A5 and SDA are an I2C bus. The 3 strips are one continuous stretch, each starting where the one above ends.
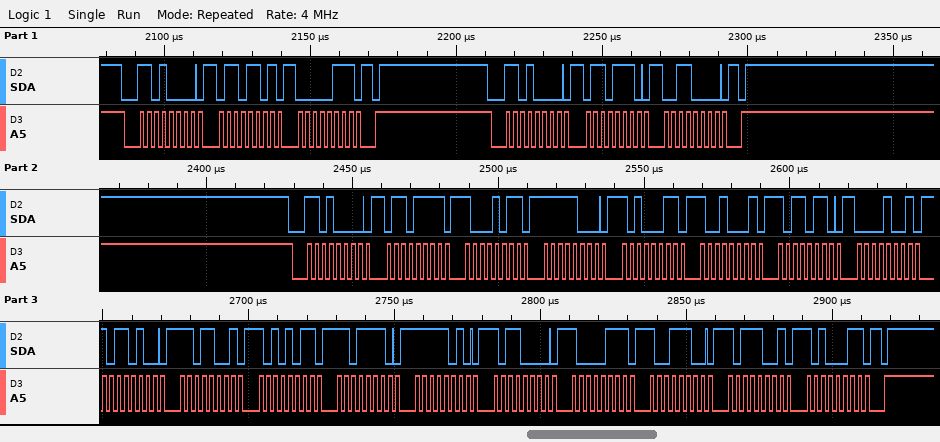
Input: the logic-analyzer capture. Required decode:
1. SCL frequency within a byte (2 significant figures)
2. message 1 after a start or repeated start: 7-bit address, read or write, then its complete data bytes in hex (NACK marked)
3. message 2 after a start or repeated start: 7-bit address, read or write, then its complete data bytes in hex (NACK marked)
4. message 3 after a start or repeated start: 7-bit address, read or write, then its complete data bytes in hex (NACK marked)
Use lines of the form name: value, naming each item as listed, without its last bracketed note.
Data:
SCL frequency within a byte: 400 kHz
message 1 after a start or repeated start: 7-bit address, read or write, then its complete data bytes in hex: 0x68 write: 6D 07
message 2 after a start or repeated start: 7-bit address, read or write, then its complete data bytes in hex: 0x68 write: 6E 30
message 3 after a start or repeated start: 7-bit address, read or write, then its complete data bytes in hex: 0x68 write: 6F 8B F8 A3 91 B6 09 B4 D9 AB DE FA B0 87 9C B9 A3
